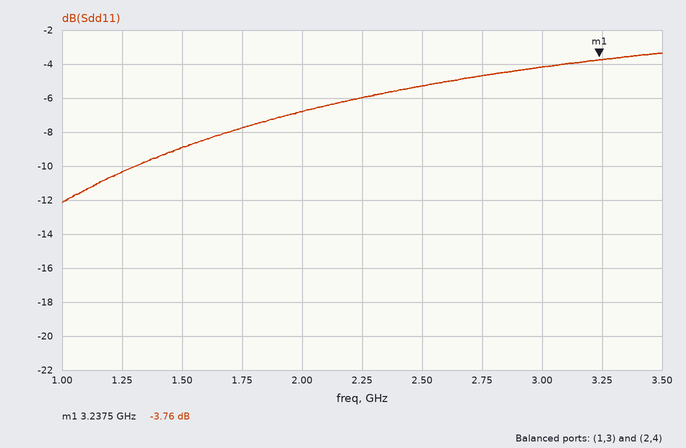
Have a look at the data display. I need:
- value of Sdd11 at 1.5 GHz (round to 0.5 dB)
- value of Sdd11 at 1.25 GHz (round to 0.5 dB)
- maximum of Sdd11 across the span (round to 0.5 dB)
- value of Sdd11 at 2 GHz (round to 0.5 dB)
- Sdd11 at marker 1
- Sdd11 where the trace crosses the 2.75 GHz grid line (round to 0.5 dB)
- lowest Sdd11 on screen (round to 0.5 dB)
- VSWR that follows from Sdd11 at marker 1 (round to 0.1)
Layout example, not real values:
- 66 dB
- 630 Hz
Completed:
- -9.0 dB
- -10.5 dB
- -3.5 dB
- -7.0 dB
- -3.76 dB
- -4.5 dB
- -12.0 dB
- 4.7
